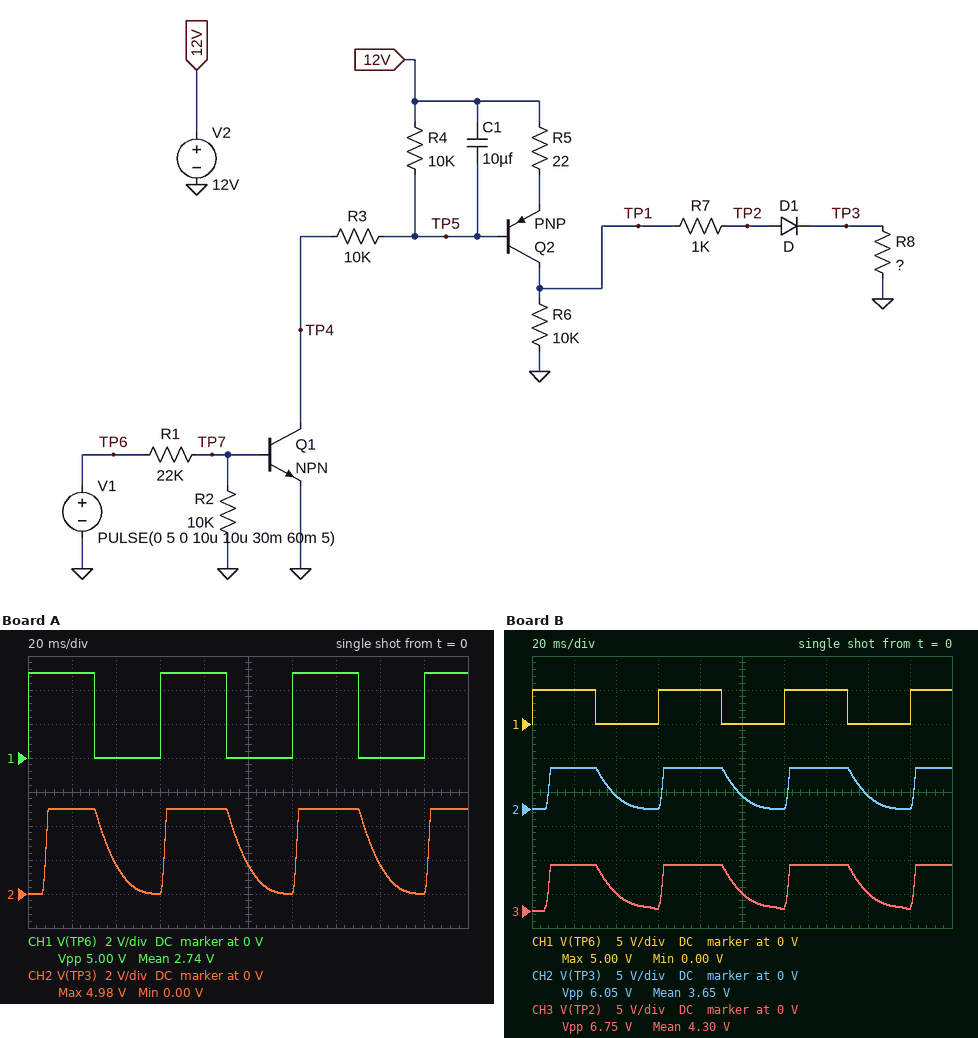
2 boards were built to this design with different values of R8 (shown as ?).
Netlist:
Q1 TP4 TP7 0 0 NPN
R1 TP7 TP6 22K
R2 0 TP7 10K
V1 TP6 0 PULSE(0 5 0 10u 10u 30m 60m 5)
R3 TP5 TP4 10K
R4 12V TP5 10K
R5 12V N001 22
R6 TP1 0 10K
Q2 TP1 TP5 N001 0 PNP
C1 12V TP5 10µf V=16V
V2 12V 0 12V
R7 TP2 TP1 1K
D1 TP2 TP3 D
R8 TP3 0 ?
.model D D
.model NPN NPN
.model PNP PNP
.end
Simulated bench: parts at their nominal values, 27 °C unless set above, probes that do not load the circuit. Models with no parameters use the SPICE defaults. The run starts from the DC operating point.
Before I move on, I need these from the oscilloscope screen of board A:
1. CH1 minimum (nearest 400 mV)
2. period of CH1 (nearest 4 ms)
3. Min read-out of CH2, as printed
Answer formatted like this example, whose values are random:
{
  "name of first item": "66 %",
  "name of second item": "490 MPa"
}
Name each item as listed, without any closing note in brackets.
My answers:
{
  "CH1 minimum": "0 V",
  "period of CH1": "60 ms",
  "Min read-out of CH2, as printed": "0.00 V"
}
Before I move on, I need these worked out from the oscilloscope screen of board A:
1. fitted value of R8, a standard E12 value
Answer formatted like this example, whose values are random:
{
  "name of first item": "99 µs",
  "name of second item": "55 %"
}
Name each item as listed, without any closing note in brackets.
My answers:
{
  "fitted value of R8, a standard E12 value": "820 Ω"
}
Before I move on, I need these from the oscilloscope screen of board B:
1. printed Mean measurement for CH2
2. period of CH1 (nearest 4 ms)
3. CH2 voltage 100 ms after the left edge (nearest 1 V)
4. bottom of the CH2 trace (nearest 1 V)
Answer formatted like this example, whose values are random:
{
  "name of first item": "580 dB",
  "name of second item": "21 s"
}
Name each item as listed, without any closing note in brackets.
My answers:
{
  "printed Mean measurement for CH2": "3.65 V",
  "period of CH1": "60 ms",
  "CH2 voltage 100 ms after the left edge": "2 V",
  "bottom of the CH2 trace": "0 V"
}
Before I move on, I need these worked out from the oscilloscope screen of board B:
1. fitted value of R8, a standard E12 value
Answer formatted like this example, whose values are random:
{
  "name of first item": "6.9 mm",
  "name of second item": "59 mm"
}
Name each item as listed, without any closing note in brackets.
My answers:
{
  "fitted value of R8, a standard E12 value": "1.2 kΩ"
}
